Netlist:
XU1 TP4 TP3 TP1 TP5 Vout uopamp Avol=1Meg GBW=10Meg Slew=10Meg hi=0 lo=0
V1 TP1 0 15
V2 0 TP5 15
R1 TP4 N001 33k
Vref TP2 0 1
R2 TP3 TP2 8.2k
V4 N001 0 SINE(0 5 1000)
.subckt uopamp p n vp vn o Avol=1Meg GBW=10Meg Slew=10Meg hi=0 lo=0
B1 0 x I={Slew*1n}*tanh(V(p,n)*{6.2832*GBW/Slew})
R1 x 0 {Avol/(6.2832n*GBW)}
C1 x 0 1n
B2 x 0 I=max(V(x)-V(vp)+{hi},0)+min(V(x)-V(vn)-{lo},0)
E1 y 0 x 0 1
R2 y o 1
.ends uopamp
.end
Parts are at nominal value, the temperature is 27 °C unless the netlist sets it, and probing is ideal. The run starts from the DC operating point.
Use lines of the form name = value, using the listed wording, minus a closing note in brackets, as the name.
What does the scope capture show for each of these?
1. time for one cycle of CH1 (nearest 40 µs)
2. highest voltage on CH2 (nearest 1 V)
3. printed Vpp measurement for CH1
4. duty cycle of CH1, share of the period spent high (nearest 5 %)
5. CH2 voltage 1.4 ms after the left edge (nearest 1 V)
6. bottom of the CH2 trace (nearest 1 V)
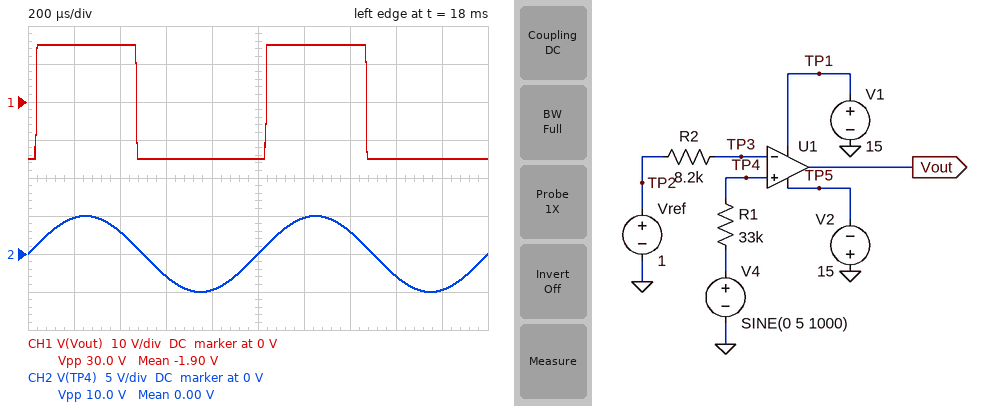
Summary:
time for one cycle of CH1 = 1.00 ms
highest voltage on CH2 = 5 V
printed Vpp measurement for CH1 = 30.0 V
duty cycle of CH1, share of the period spent high = 45 %
CH2 voltage 1.4 ms after the left edge = 3 V
bottom of the CH2 trace = -5 V
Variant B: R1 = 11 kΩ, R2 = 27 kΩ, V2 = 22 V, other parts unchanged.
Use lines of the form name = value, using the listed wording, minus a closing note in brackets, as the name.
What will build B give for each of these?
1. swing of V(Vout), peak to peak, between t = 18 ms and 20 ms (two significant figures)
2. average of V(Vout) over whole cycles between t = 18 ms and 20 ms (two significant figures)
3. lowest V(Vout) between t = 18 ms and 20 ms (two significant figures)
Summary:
swing of V(Vout), peak to peak, between t = 18 ms and 20 ms = 37 V
average of V(Vout) over whole cycles between t = 18 ms and 20 ms = -5.9 V
lowest V(Vout) between t = 18 ms and 20 ms = -22 V
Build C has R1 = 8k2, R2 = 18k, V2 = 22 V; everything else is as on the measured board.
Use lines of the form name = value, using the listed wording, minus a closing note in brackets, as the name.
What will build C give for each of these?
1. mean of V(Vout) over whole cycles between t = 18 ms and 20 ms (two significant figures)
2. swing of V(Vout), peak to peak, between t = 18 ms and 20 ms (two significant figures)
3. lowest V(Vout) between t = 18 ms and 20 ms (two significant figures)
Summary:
mean of V(Vout) over whole cycles between t = 18 ms and 20 ms = -5.9 V
swing of V(Vout), peak to peak, between t = 18 ms and 20 ms = 37 V
lowest V(Vout) between t = 18 ms and 20 ms = -22 V
